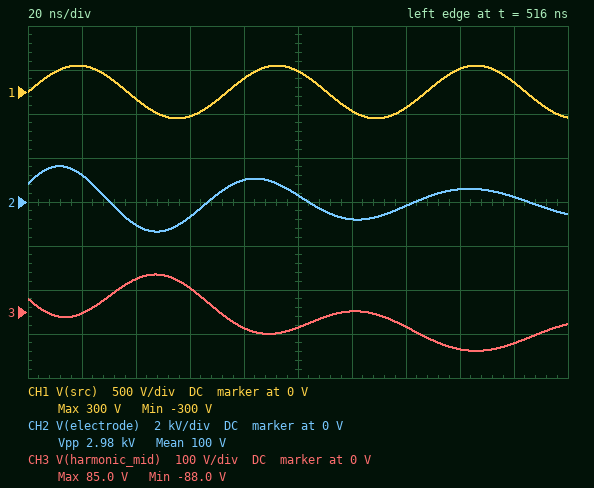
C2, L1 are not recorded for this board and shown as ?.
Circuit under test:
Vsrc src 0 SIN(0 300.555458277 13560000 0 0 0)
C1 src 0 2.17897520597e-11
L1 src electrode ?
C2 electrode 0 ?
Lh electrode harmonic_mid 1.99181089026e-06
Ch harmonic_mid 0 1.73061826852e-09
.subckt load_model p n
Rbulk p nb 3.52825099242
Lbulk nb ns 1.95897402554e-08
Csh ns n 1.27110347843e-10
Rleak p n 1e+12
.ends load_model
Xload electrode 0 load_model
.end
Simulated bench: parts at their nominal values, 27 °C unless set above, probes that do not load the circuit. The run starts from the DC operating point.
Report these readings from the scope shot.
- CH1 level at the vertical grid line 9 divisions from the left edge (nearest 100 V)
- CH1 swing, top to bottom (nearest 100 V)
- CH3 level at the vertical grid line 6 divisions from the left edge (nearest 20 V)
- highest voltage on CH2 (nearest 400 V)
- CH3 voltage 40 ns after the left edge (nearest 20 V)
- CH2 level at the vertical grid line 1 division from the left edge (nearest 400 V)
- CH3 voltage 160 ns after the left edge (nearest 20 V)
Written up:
100 V
600 V
0 V
1.6 kV
80 V
1.2 kV
-80 V
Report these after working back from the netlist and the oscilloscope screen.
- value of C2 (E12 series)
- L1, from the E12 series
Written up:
270 pF
330 nH
